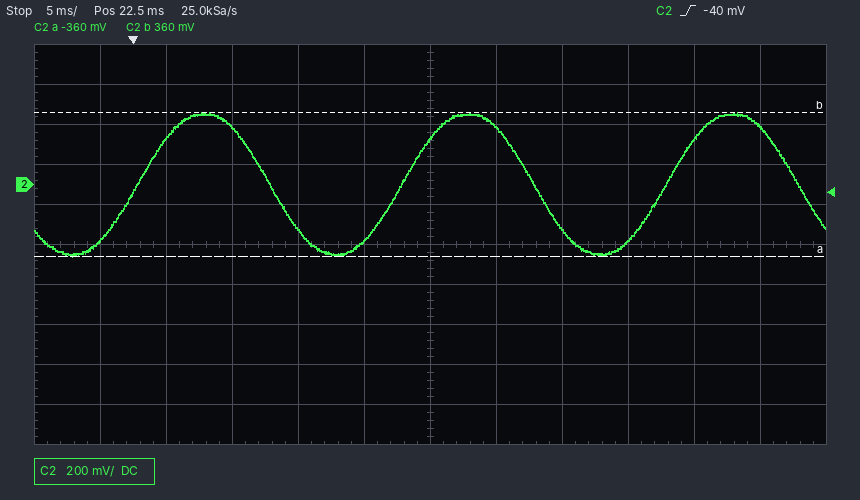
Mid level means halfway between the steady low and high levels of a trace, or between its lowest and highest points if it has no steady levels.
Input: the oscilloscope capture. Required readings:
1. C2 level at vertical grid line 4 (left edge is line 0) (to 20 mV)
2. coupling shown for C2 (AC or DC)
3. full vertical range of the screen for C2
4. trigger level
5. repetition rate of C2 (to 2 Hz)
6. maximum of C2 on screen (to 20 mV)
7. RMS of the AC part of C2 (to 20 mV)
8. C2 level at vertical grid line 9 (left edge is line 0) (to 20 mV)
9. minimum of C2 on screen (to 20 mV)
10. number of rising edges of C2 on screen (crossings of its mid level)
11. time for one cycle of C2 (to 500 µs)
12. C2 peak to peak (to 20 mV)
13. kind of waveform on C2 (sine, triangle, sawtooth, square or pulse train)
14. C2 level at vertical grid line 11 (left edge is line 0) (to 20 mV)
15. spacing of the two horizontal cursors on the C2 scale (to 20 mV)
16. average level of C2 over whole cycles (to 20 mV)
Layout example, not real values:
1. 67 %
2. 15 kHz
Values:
1. -220 mV
2. DC
3. 2 V
4. -40 mV
5. 50 Hz
6. 360 mV
7. 260 mV
8. -280 mV
9. -360 mV
10. 3
11. 20.0 ms
12. 720 mV
13. sine
14. 280 mV
15. 720 mV
16. 0 mV
